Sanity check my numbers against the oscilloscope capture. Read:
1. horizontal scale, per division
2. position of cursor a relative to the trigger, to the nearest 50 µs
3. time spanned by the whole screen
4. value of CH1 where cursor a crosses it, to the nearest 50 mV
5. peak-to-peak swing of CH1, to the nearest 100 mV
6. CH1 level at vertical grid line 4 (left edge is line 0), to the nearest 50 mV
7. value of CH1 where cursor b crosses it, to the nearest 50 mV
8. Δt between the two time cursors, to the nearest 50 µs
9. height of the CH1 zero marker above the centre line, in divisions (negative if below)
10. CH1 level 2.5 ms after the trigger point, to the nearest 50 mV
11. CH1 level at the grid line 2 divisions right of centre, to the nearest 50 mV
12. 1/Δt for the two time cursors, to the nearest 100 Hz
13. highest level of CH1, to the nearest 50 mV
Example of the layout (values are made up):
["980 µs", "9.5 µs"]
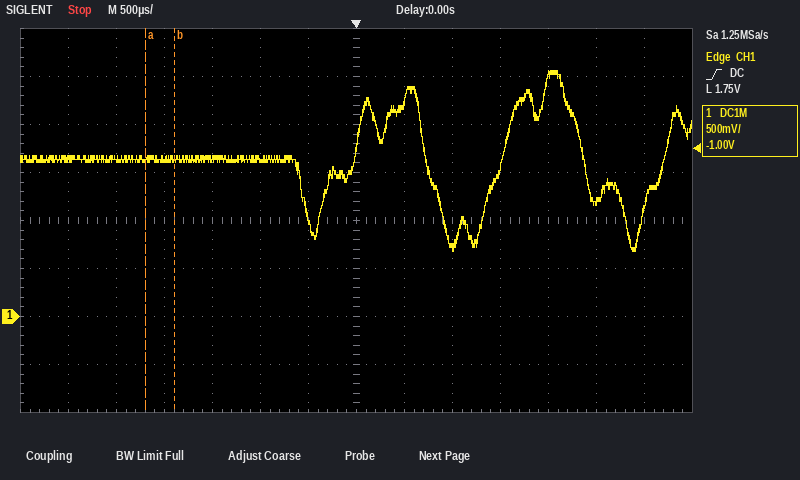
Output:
["500 µs", "-2.20 ms", "7 ms", "1.65 V", "1.90 V", "1.65 V", "1.65 V", "300 µs", "-2.0 div", "1.20 V", "700 mV", "3.3 kHz", "2.55 V"]
